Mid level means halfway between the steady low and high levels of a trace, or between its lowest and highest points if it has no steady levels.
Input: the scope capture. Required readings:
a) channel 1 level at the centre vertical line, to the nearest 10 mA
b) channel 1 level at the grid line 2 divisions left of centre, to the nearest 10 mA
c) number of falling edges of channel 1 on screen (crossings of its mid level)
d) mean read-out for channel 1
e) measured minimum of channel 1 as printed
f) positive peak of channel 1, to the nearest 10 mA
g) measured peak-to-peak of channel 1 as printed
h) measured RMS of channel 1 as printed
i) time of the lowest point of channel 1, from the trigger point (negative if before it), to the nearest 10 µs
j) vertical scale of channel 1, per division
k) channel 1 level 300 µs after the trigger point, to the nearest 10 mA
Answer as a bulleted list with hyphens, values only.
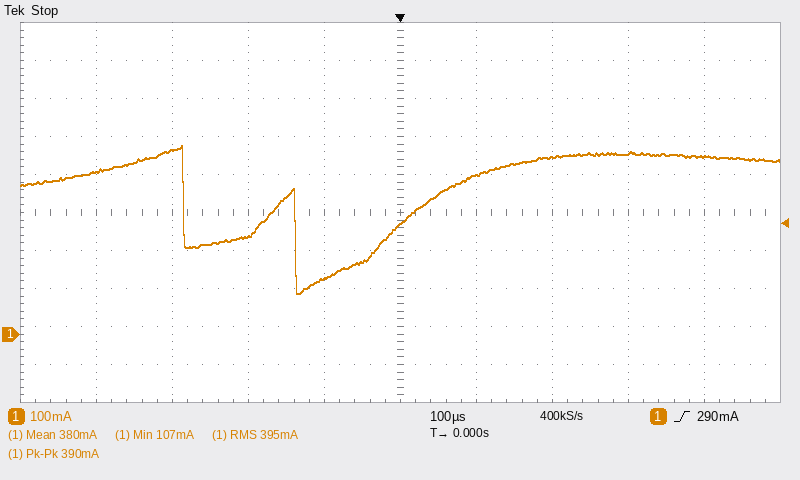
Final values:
- 290 mA
- 260 mA
- 2
- 380 mA
- 107 mA
- 500 mA
- 390 mA
- 395 mA
- -130 µs
- 100 mA
- 480 mA
